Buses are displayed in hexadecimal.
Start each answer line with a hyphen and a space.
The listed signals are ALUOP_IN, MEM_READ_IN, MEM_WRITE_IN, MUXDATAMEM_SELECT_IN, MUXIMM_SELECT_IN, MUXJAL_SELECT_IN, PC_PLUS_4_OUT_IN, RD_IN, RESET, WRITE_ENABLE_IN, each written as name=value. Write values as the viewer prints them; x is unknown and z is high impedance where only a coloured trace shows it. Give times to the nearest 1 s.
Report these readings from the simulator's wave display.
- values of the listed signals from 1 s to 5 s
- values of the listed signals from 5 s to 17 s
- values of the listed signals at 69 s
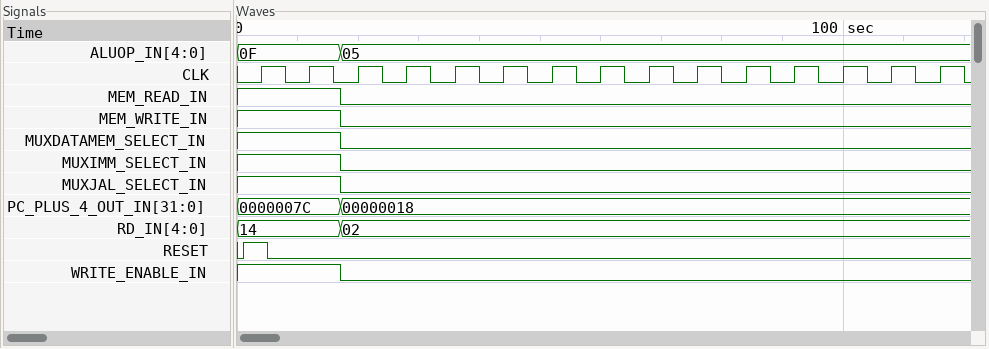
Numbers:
- ALUOP_IN=0F, MEM_READ_IN=1, MEM_WRITE_IN=1, MUXDATAMEM_SELECT_IN=1, MUXIMM_SELECT_IN=1, MUXJAL_SELECT_IN=1, PC_PLUS_4_OUT_IN=0000007C, RD_IN=14, RESET=1, WRITE_ENABLE_IN=1
- ALUOP_IN=0F, MEM_READ_IN=1, MEM_WRITE_IN=1, MUXDATAMEM_SELECT_IN=1, MUXIMM_SELECT_IN=1, MUXJAL_SELECT_IN=1, PC_PLUS_4_OUT_IN=0000007C, RD_IN=14, RESET=0, WRITE_ENABLE_IN=1
- ALUOP_IN=05, MEM_READ_IN=0, MEM_WRITE_IN=0, MUXDATAMEM_SELECT_IN=0, MUXIMM_SELECT_IN=0, MUXJAL_SELECT_IN=0, PC_PLUS_4_OUT_IN=00000018, RD_IN=02, RESET=0, WRITE_ENABLE_IN=0
